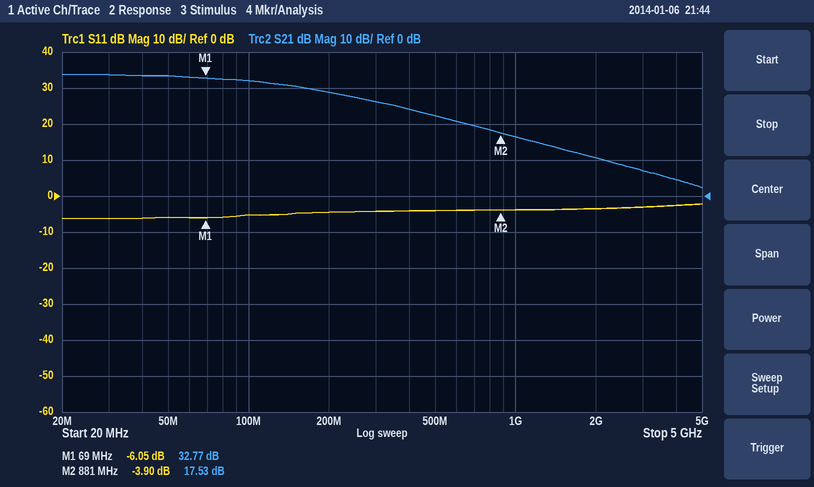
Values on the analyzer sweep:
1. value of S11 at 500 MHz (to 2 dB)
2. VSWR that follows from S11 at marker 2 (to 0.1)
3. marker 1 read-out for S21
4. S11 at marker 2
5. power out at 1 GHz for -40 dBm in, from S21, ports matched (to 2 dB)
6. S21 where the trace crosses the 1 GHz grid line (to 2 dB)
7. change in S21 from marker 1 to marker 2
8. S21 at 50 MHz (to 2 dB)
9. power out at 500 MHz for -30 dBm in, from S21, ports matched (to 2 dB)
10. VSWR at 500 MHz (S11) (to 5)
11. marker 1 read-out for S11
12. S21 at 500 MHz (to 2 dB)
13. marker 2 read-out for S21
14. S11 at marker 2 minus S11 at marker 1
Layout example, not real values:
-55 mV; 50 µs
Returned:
-4 dB; 4.5; 32.77 dB; -3.90 dB; -24 dBm; 16 dB; -15.24 dB; 34 dB; -8 dBm; 5; -6.05 dB; 22 dB; 17.53 dB; 2.15 dB
